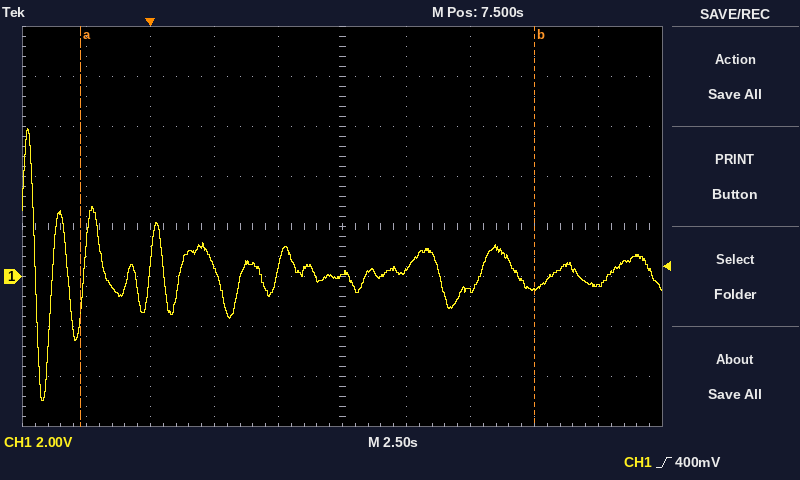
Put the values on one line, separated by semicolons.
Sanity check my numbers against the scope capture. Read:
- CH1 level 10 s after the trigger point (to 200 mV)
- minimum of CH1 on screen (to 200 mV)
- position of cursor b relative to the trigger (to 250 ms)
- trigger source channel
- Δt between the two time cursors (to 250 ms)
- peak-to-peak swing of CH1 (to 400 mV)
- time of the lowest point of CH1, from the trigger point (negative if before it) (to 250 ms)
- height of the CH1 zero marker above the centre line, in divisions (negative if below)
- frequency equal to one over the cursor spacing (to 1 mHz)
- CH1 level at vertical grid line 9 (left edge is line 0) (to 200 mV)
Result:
200 mV; -5.0 V; +15.00 s; CH1; 17.75 s; 10.8 V; -4.25 s; -1.0 div; 56 mHz; -400 mV
